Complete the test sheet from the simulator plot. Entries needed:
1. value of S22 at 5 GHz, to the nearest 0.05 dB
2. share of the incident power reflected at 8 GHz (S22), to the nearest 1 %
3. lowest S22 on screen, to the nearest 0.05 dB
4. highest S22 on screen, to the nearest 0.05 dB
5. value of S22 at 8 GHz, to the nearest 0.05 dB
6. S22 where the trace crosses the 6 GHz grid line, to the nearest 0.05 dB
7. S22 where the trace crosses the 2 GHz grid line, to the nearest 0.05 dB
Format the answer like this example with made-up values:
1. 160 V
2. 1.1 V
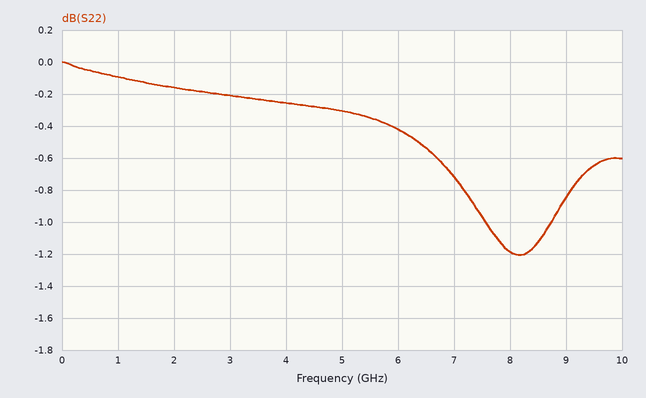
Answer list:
1. -0.30 dB
2. 76 %
3. -1.20 dB
4. 0.00 dB
5. -1.20 dB
6. -0.40 dB
7. -0.15 dB
